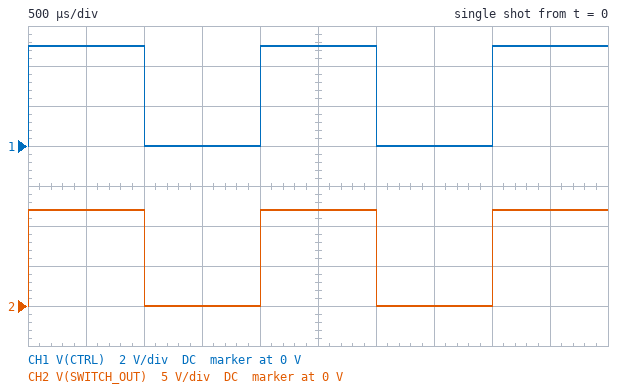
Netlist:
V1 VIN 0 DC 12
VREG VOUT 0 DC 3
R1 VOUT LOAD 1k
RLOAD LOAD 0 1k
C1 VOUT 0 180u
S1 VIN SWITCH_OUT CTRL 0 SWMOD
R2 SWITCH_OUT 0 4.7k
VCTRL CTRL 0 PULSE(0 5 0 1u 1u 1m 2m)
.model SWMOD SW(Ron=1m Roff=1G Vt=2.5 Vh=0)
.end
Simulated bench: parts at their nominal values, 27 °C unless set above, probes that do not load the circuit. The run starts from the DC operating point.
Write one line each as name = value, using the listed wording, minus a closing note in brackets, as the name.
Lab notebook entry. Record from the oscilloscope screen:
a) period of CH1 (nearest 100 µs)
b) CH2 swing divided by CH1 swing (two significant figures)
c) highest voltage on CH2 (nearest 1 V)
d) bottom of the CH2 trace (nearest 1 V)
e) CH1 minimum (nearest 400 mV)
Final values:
period of CH1 = 2.0 ms
CH2 swing divided by CH1 swing = 2.4
highest voltage on CH2 = 12 V
bottom of the CH2 trace = 0 V
CH1 minimum = 0 V
